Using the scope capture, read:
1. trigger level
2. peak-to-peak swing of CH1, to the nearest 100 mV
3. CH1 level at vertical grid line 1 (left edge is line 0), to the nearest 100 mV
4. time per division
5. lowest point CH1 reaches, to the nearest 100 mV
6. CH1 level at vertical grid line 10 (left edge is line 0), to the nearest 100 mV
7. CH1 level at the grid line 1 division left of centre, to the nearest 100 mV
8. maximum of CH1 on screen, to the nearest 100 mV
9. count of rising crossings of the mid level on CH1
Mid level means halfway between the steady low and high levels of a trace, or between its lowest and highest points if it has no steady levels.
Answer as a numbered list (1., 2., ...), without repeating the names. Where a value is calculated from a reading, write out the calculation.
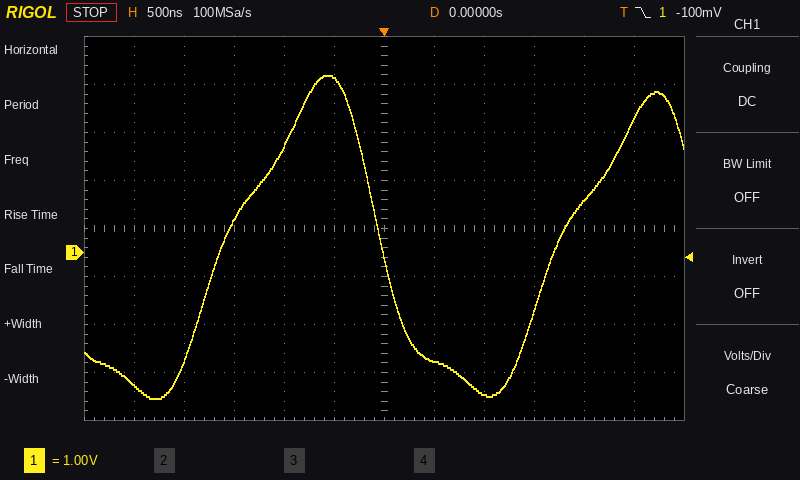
1. -100 mV
2. 3.7 V − (-3.0 V) = 6.7 V
3. -2.8 V
4. 500 ns
5. -3.0 V
6. 1.1 V
7. 3.6 V
8. 3.7 V
9. 2
